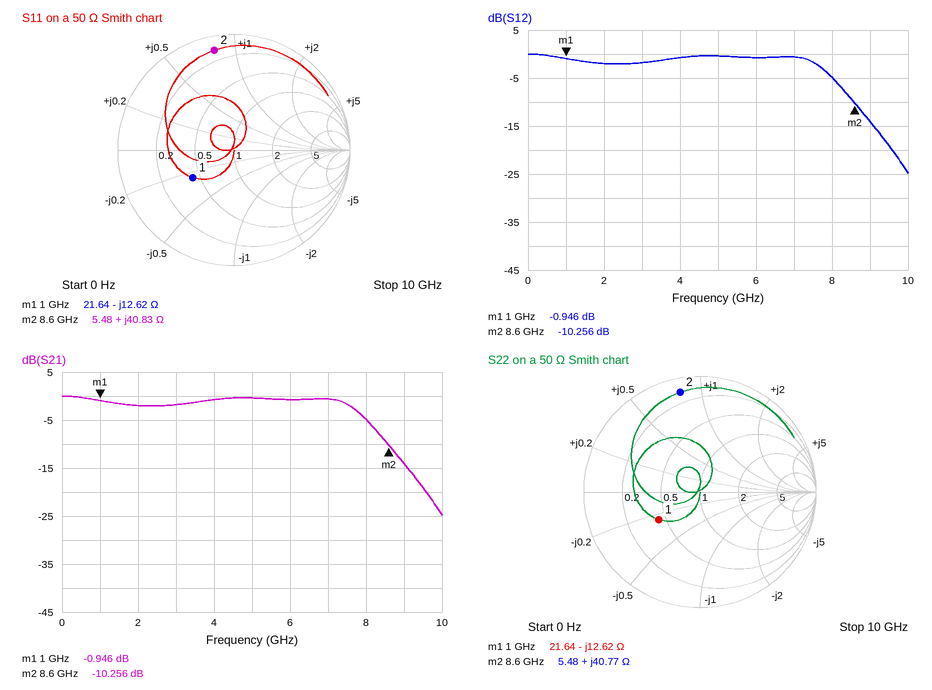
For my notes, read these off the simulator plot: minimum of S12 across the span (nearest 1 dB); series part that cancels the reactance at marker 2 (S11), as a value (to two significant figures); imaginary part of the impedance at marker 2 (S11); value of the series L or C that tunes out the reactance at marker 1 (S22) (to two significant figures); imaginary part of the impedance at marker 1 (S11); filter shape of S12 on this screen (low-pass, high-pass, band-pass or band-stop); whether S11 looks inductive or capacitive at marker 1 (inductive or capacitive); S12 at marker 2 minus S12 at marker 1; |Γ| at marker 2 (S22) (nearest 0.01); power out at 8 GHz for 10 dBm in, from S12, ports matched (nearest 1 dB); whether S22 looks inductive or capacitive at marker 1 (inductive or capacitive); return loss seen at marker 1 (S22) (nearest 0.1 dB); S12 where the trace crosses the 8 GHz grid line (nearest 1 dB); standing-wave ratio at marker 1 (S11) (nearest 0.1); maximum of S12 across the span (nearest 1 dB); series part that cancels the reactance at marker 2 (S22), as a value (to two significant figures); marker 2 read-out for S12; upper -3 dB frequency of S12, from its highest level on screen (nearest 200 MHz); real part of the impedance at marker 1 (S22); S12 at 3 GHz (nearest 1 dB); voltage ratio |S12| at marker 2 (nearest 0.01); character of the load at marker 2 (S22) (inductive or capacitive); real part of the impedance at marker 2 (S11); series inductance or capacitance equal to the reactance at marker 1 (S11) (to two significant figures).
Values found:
-25 dB
450 fF
+40.83 Ω
2.0 nH
-12.62 Ω
low-pass
capacitive
-9.310 dB
0.88
5 dBm
capacitive
7.4 dB
-5 dB
2.5
0 dB
450 fF
-10.256 dB
7.8 GHz
21.64 Ω
-2 dB
0.31
inductive
5.48 Ω
13 pF
